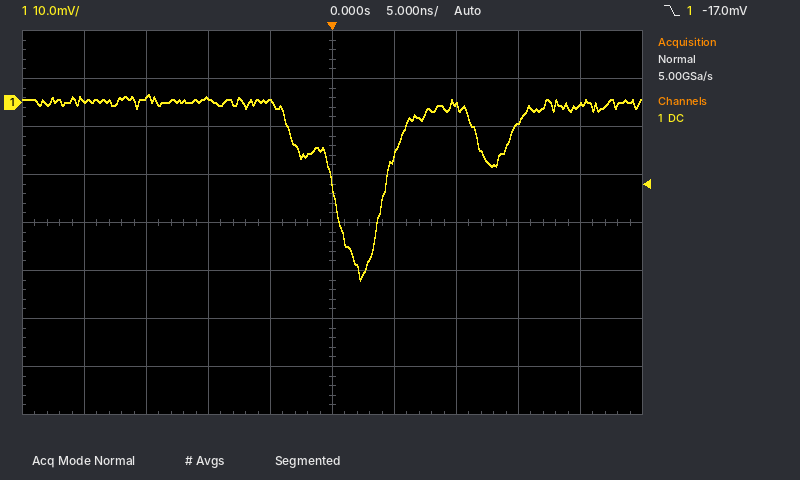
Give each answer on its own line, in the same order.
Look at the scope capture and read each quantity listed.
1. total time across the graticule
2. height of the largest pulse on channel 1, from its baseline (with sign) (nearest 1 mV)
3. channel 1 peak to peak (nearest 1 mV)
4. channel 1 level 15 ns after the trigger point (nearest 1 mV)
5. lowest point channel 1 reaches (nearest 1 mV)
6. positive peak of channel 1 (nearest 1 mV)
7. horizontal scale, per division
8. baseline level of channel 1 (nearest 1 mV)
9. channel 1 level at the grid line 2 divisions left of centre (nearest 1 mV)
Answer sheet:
50 ns
-37 mV
39 mV
-4 mV
-37 mV
2 mV
5 ns
0 mV
1 mV
